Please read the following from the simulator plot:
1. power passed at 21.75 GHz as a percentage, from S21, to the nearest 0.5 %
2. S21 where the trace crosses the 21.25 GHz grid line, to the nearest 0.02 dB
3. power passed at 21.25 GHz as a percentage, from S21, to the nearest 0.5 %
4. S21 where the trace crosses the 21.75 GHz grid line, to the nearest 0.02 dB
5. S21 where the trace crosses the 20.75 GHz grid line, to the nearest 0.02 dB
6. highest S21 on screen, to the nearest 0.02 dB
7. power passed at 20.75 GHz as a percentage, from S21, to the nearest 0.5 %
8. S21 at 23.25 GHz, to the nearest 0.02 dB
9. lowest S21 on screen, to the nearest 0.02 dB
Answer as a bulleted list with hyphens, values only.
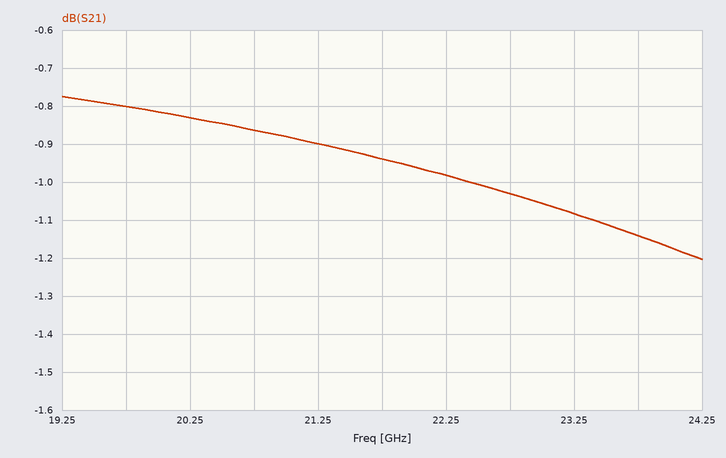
- 80.5 %
- -0.90 dB
- 81.5 %
- -0.94 dB
- -0.86 dB
- -0.78 dB
- 82.0 %
- -1.08 dB
- -1.20 dB
